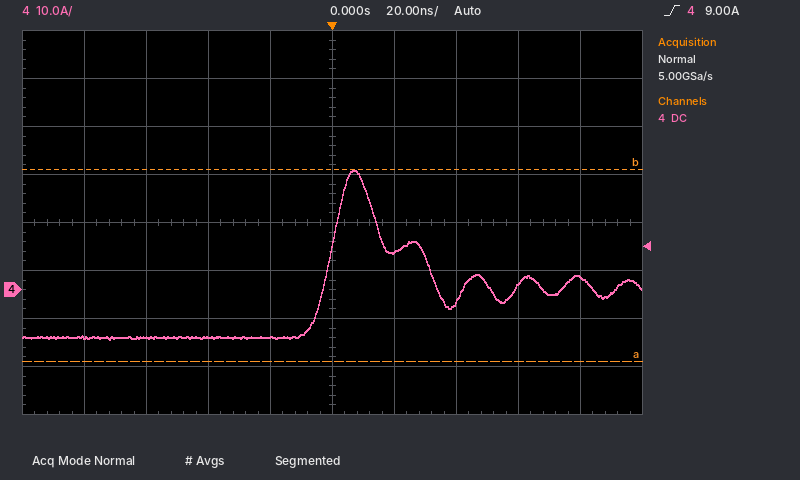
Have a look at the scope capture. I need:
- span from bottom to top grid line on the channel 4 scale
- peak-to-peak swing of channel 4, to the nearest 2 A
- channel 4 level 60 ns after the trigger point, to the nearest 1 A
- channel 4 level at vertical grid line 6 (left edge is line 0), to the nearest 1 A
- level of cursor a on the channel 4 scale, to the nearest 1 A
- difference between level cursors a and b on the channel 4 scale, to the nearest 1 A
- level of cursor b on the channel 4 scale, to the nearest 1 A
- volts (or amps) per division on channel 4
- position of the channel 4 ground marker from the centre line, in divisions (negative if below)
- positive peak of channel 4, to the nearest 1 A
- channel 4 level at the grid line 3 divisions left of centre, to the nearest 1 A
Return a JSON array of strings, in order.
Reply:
["80 A", "36 A", "1 A", "8 A", "-15 A", "40 A", "25 A", "10 A", "-1.4 div", "25 A", "-10 A"]
